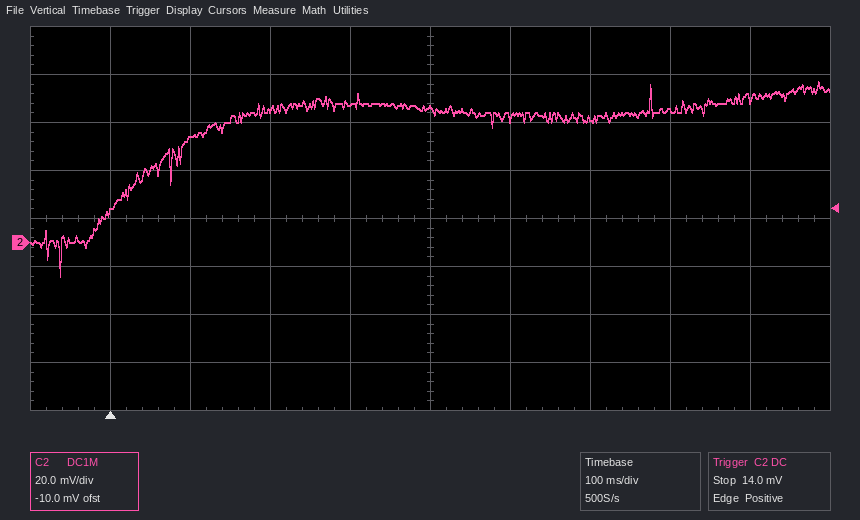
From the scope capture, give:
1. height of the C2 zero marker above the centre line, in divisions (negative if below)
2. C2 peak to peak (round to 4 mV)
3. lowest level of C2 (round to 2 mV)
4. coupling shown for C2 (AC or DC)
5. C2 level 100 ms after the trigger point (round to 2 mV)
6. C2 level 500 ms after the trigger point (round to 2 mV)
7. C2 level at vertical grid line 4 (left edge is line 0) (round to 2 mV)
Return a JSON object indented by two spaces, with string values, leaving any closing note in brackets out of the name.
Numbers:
{
  "height of the C2 zero marker above the centre line, in divisions": "-0.5 div",
  "C2 peak to peak": "80 mV",
  "lowest level of C2": "-14 mV",
  "coupling shown for C2": "DC",
  "C2 level 100 ms after the trigger point": "44 mV",
  "C2 level 500 ms after the trigger point": "52 mV",
  "C2 level at vertical grid line 4 (left edge is line 0)": "58 mV"
}
